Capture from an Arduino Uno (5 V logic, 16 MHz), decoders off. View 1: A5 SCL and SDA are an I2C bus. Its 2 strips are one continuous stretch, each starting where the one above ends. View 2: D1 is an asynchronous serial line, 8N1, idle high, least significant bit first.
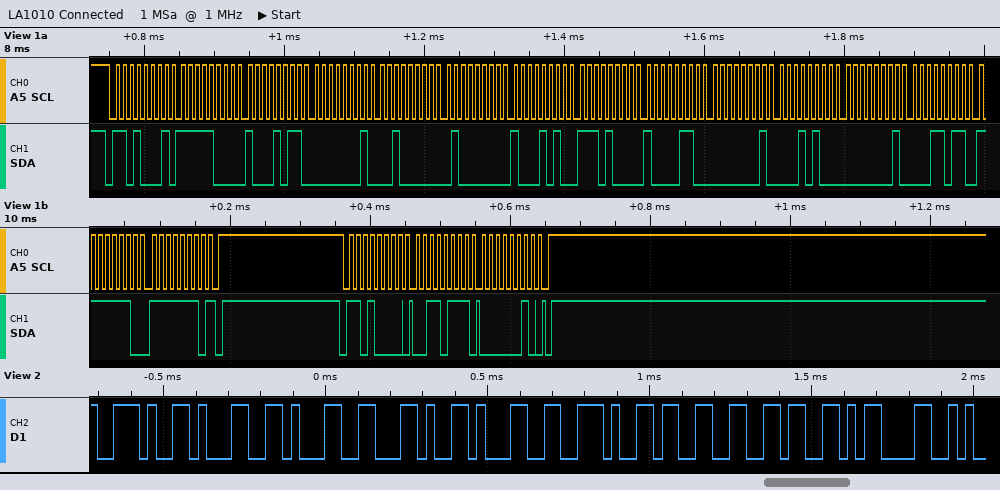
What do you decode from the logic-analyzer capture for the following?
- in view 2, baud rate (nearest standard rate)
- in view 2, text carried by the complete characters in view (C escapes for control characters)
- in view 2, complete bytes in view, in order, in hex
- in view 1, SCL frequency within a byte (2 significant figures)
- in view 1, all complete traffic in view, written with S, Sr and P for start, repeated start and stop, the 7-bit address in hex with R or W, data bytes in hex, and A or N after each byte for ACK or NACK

38400 baud
".11,1.36\r"
2E 31 31 2C 31 2E 33 36 0D
100 kHz
S 68R A F8 A 8B A 01 A 20 A 40 A 8A A E8 A 86 A 01 A 14 A 01 A 1B A FE A FE N P S 68W A 37 A 02 A P
